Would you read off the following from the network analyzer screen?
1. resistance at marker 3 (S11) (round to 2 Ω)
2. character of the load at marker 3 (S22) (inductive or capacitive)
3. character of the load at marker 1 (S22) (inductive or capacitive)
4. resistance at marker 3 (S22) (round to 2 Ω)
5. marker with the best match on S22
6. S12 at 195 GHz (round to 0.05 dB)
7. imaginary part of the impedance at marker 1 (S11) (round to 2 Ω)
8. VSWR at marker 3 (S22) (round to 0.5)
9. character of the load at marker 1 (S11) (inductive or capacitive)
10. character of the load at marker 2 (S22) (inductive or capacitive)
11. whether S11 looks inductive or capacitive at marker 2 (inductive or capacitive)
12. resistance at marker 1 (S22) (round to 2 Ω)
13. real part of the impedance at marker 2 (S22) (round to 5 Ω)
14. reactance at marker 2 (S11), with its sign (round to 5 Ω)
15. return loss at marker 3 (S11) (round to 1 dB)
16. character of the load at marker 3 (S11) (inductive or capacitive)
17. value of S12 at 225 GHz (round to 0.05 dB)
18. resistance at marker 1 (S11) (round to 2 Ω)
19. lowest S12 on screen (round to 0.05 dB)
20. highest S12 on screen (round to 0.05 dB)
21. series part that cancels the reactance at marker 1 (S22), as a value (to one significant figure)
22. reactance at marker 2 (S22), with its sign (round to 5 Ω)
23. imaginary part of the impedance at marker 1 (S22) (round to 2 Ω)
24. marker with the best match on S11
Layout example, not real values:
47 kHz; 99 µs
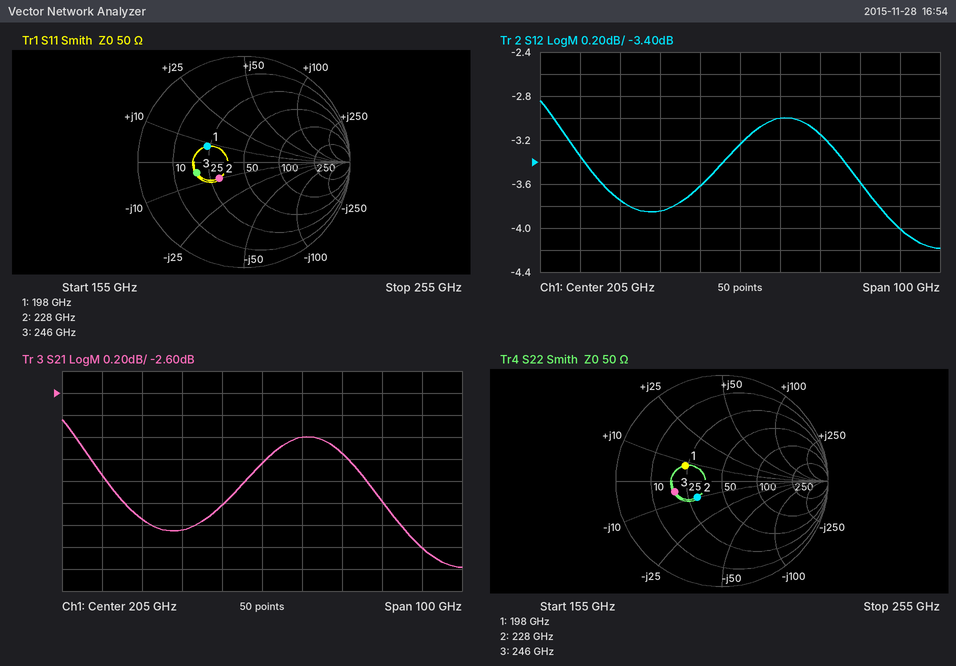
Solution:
18 Ω; capacitive; inductive; 18 Ω; marker 2; -3.60 dB; +8 Ω; 2.5; inductive; capacitive; capacitive; 24 Ω; 30 Ω; -10 Ω; 7 dB; capacitive; -3.15 dB; 24 Ω; -4.20 dB; -2.85 dB; 100 fF; -10 Ω; +8 Ω; marker 2
